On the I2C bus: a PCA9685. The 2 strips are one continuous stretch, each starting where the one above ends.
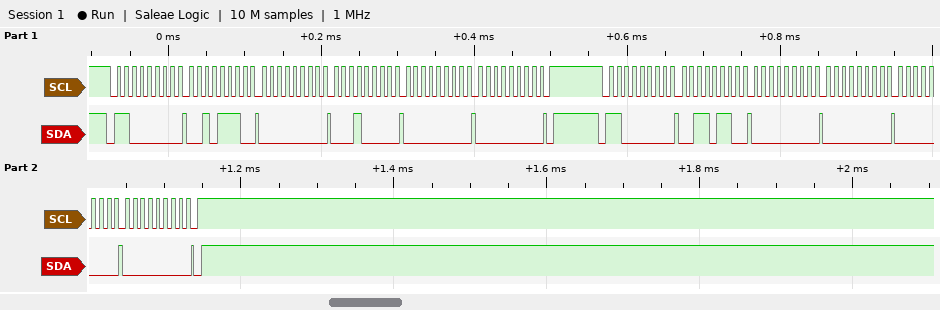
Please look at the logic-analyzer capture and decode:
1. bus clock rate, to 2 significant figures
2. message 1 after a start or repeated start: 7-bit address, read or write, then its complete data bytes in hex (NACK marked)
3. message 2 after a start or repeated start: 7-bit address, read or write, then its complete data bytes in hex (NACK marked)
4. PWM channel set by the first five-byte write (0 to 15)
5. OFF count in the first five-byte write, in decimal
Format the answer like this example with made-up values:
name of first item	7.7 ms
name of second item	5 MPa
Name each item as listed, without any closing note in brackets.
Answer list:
bus clock rate, to 2 significant figures	100 kHz
message 1 after a start or repeated start: 7-bit address, read or write, then its complete data bytes in hex	0x60 write: 2E 00 10 00 00
message 2 after a start or repeated start: 7-bit address, read or write, then its complete data bytes in hex	0x60 write: 36 00 00 00 00
PWM channel set by the first five-byte write	10
OFF count in the first five-byte write, in decimal	0
